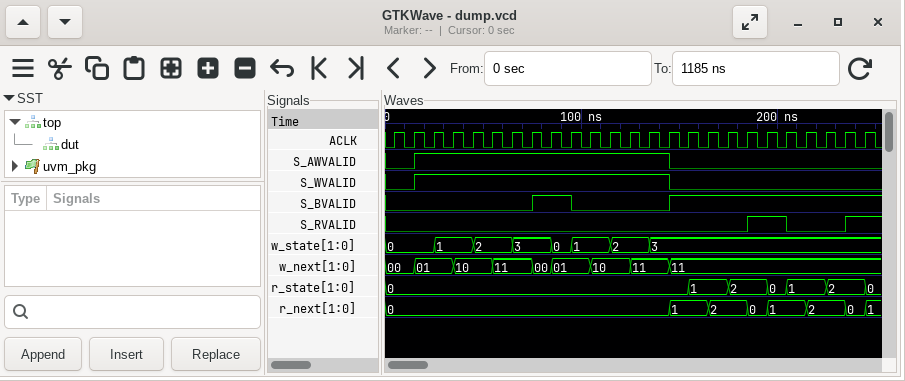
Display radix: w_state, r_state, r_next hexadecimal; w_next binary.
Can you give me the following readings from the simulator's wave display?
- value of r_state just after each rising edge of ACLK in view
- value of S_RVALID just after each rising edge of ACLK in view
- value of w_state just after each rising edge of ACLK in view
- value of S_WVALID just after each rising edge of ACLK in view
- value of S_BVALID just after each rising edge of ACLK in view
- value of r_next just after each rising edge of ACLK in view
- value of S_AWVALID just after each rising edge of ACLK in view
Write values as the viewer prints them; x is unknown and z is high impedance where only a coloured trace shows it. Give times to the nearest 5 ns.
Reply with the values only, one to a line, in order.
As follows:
0, 0, 0, 0, 0, 0, 0, 0, 0, 0, 0, 0, 0, 0, 0, 1, 1, 2, 2, 0, 1, 1, 2, 2, 0
0 0 0 0 0 0 0 0 0 0 0 0 0 0 0 0 0 0 1 1 0 0 0 1 1
0, 0, 1, 1, 2, 2, 3, 3, 0, 1, 1, 2, 2, 3, 3, 3, 3, 3, 3, 3, 3, 3, 3, 3, 3
0 1 1 1 1 1 1 1 1 1 1 1 1 1 0 0 0 0 0 0 0 0 0 0 0
0 0 0 0 0 0 0 1 1 0 0 0 0 0 1 1 1 1 1 1 1 1 1 1 1
0, 0, 0, 0, 0, 0, 0, 0, 0, 0, 0, 0, 0, 0, 1, 1, 2, 2, 0, 1, 1, 2, 2, 0, 1
0 1 1 1 1 1 1 1 1 1 1 1 1 1 0 0 0 0 0 0 0 0 0 0 0
